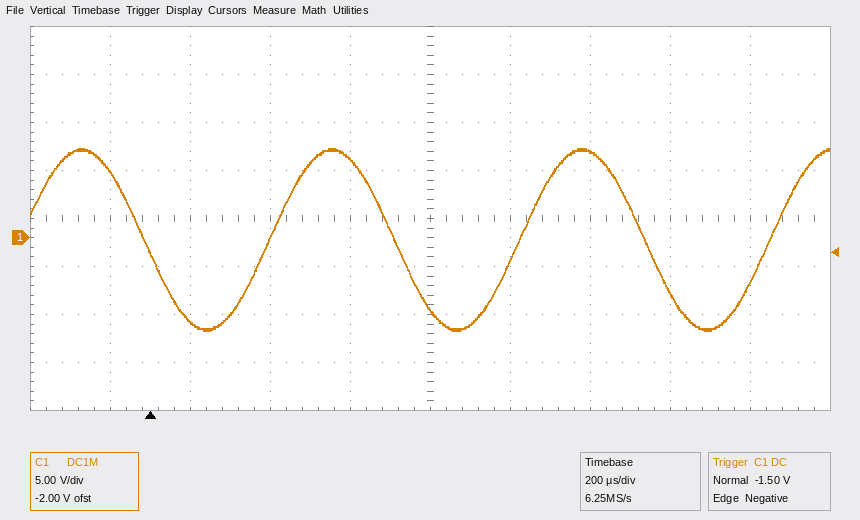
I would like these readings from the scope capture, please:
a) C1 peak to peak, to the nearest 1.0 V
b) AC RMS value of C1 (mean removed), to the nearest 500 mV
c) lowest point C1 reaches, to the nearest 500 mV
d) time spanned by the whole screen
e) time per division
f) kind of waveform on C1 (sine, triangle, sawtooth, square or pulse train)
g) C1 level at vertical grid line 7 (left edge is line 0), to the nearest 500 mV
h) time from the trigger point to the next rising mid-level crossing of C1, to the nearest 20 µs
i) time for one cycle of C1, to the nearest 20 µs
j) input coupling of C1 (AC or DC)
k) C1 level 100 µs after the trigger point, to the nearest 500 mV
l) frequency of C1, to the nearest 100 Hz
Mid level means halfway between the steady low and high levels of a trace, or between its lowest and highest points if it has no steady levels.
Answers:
19.0 V
6.5 V
-9.5 V
2 ms
200 µs
sine
9.0 V
300 µs
620 µs
DC
-8.5 V
1.6 kHz
